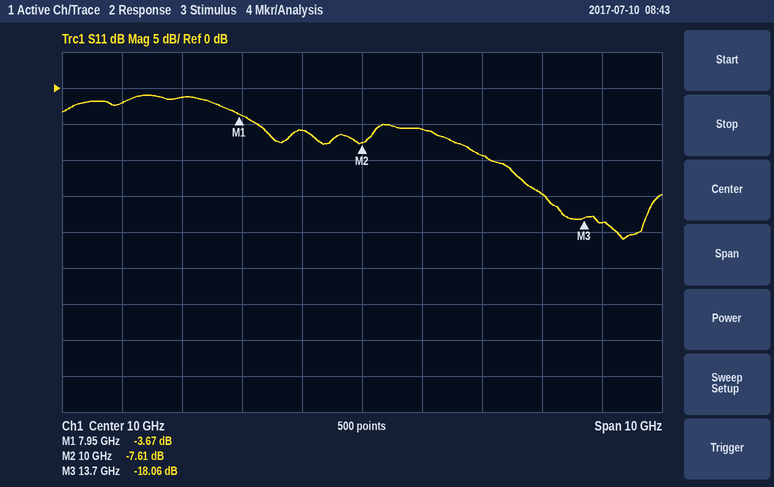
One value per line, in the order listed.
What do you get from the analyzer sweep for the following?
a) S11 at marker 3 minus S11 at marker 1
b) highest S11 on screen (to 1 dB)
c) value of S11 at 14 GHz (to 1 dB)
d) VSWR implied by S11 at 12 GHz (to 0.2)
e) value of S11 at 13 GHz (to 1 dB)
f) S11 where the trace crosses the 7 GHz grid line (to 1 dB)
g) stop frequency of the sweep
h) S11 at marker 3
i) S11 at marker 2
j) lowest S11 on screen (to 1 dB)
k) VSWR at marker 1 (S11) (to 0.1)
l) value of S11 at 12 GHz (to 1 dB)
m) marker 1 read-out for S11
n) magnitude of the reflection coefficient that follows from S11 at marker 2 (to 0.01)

-14.39 dB
-1 dB
-19 dB
2.0
-15 dB
-1 dB
15 GHz
-18.06 dB
-7.61 dB
-21 dB
4.8
-9 dB
-3.67 dB
0.42
